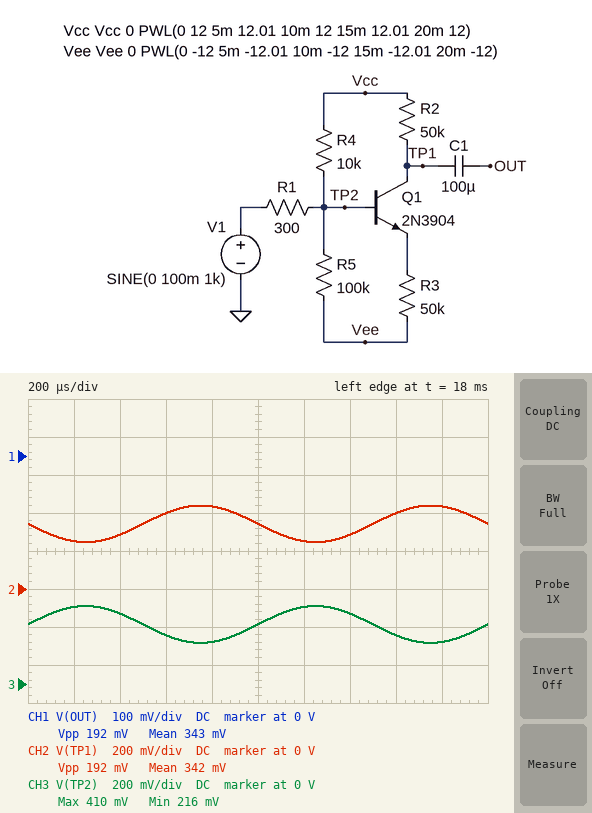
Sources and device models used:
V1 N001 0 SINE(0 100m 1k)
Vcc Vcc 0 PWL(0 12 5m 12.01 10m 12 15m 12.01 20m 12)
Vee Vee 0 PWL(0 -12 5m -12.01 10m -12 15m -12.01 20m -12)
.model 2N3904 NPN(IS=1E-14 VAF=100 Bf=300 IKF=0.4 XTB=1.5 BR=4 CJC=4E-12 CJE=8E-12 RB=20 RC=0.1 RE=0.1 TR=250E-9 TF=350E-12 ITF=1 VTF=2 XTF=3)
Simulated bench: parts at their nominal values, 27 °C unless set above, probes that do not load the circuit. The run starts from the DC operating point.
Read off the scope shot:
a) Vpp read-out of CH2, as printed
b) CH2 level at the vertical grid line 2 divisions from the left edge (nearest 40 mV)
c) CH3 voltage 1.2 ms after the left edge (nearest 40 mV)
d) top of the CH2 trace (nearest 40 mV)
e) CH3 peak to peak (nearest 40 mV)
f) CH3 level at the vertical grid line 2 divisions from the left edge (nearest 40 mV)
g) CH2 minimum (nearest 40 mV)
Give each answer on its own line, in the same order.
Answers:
192 mV
280 mV
400 mV
440 mV
200 mV
360 mV
240 mV
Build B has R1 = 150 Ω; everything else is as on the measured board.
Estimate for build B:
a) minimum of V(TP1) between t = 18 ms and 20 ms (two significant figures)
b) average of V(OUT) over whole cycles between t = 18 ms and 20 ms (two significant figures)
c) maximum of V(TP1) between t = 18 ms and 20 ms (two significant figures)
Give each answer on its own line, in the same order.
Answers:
400 mV
500 mV
590 mV
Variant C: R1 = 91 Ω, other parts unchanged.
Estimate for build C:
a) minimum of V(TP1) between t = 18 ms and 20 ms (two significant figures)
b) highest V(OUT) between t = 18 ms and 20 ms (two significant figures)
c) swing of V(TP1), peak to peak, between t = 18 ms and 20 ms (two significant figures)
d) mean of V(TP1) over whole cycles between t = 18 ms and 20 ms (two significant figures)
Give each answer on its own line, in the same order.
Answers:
460 mV
660 mV
200 mV
560 mV
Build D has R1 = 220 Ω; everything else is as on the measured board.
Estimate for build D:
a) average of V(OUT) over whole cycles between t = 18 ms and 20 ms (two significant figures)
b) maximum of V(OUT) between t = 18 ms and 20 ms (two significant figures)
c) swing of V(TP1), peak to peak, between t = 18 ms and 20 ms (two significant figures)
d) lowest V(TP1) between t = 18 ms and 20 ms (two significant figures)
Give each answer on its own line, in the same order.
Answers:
420 mV
520 mV
190 mV
330 mV
